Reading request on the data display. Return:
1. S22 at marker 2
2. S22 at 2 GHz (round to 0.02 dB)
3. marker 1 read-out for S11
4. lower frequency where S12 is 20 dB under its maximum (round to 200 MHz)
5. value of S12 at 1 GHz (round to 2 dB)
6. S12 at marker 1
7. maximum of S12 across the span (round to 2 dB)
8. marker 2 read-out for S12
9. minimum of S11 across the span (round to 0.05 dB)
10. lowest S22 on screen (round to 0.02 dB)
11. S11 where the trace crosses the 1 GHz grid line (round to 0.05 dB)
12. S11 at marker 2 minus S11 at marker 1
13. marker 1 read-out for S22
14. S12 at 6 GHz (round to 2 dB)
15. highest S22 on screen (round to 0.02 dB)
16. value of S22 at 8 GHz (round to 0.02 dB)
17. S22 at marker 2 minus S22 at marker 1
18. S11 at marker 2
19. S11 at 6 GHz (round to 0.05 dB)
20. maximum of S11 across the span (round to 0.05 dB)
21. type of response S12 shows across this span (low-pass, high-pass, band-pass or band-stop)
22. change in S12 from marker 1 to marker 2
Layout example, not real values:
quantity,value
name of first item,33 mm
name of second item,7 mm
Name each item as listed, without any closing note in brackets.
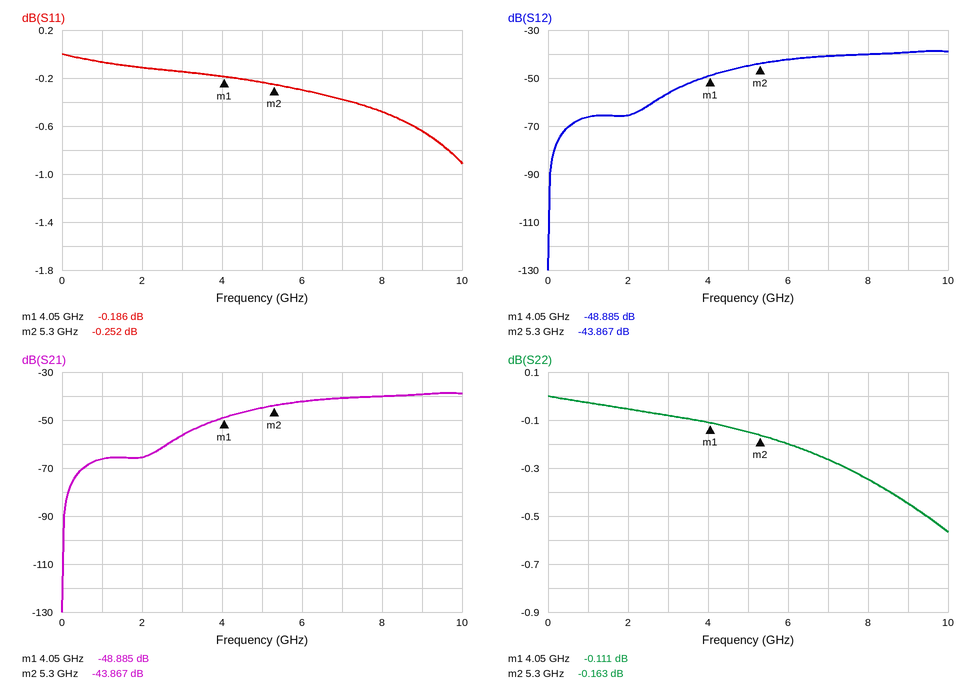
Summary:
quantity,value
S22 at marker 2,-0.163 dB
S22 at 2 GHz,-0.06 dB
marker 1 read-out for S11,-0.186 dB
lower frequency where S12 is 20 dB under its maximum,2.8 GHz
value of S12 at 1 GHz,-66 dB
S12 at marker 1,-48.885 dB
maximum of S12 across the span,-38 dB
marker 2 read-out for S12,-43.867 dB
minimum of S11 across the span,-0.90 dB
lowest S22 on screen,-0.56 dB
S11 where the trace crosses the 1 GHz grid line,-0.05 dB
S11 at marker 2 minus S11 at marker 1,-0.066 dB
marker 1 read-out for S22,-0.111 dB
S12 at 6 GHz,-42 dB
highest S22 on screen,0.00 dB
value of S22 at 8 GHz,-0.34 dB
S22 at marker 2 minus S22 at marker 1,-0.052 dB
S11 at marker 2,-0.252 dB
S11 at 6 GHz,-0.30 dB
maximum of S11 across the span,0.00 dB
type of response S12 shows across this span,high-pass
change in S12 from marker 1 to marker 2,5.018 dB
